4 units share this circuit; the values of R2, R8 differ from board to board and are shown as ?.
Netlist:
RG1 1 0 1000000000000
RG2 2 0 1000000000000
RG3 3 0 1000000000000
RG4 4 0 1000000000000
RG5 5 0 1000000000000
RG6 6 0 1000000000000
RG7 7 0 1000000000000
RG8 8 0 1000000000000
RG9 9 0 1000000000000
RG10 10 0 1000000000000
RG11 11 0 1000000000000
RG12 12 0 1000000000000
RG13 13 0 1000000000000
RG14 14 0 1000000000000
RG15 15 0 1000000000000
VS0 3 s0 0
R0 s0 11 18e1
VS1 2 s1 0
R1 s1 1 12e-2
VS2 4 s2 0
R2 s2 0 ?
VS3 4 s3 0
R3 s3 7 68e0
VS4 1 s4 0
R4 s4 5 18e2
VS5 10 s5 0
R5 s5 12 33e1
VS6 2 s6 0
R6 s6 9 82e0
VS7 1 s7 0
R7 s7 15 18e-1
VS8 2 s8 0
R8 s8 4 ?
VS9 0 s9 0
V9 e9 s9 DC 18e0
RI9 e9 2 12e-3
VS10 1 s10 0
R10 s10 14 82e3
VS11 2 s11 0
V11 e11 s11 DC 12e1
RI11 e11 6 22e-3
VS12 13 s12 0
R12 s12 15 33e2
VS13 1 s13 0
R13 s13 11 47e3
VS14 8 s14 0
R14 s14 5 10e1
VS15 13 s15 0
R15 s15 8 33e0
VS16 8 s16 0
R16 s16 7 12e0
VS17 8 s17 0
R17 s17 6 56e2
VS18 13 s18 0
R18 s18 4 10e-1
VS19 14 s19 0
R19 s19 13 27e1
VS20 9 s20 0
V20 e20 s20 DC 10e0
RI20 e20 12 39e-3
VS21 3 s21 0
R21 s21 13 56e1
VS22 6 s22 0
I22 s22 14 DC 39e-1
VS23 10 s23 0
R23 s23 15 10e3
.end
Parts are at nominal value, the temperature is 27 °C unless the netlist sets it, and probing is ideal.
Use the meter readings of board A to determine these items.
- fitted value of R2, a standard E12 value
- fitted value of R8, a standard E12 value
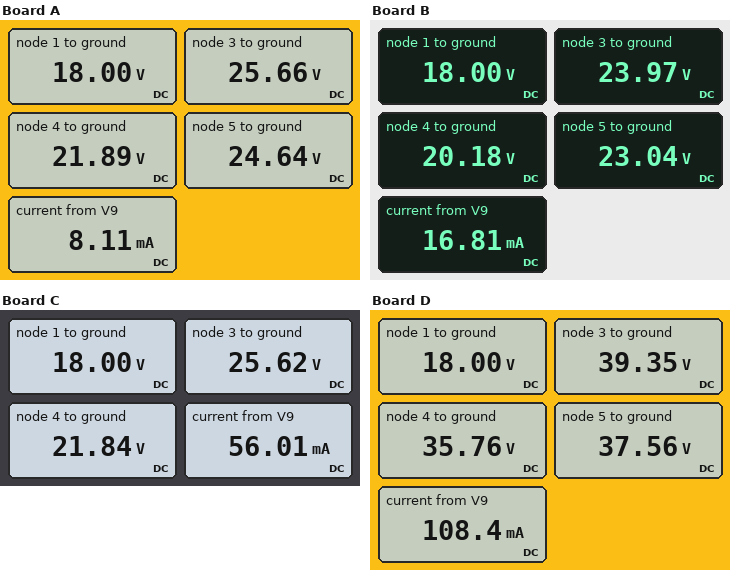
2.7 kΩ
1 Ω
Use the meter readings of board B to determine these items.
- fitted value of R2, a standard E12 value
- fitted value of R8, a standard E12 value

1.2 kΩ
0.56 Ω
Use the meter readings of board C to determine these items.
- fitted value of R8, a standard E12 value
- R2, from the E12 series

1 Ω
390 Ω
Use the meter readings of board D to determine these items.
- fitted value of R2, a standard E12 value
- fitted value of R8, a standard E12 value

330 Ω
4.7 Ω
